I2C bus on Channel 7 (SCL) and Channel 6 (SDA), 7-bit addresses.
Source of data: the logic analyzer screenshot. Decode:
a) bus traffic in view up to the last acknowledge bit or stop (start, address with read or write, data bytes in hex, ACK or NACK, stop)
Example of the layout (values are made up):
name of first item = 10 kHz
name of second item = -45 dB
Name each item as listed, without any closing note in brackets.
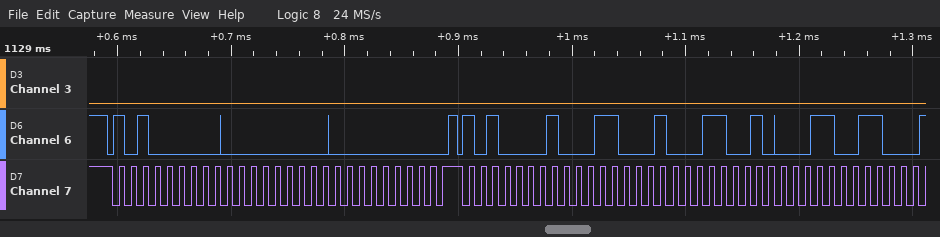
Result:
bus traffic in view up to the last acknowledge bit or stop = start, address 50 write ACK, 00 ACK, 00 ACK, stop, start, address 50 read ACK, 31 ACK, 32 ACK, 33 ACK
